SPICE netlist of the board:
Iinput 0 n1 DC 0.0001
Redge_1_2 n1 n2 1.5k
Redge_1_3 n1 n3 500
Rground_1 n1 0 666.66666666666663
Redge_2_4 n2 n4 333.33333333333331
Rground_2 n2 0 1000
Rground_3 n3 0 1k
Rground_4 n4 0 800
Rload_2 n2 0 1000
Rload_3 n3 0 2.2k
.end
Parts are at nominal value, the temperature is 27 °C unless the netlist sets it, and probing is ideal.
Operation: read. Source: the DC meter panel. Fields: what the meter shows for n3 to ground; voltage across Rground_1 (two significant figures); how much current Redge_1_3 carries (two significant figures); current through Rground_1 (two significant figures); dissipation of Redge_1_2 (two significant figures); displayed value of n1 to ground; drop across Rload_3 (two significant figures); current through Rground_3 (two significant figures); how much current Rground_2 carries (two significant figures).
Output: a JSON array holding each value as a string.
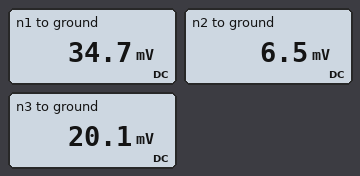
["20.1 mV", "35 mV", "29 µA", "52 µA", "530 nW", "34.7 mV", "20 mV", "20 µA", "6.5 µA"]
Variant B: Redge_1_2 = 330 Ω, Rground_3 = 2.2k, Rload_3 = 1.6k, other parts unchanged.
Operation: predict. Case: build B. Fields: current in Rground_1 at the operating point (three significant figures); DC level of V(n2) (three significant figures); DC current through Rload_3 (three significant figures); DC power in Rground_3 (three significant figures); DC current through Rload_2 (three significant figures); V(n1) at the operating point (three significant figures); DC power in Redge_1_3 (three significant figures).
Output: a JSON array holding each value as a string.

["40.8 µA", "13.9 mV", "11.0 µA", "142 nW", "13.9 µA", "27.2 mV", "182 nW"]
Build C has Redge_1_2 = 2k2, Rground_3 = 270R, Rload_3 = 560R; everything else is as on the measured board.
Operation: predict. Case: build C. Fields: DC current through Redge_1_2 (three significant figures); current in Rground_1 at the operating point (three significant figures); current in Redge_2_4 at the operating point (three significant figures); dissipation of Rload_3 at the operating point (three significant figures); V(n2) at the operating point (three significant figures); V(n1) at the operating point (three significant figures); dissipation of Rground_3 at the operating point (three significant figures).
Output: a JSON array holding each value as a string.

["11.7 µA", "44.7 µA", "3.58 µA", "113 nW", "4.06 mV", "29.8 mV", "234 nW"]
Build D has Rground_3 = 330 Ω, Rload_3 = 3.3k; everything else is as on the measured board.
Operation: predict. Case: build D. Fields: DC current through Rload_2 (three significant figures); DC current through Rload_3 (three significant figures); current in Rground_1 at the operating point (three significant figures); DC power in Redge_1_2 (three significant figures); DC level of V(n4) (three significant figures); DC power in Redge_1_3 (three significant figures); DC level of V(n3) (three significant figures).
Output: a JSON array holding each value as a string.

["5.71 µA", "3.45 µA", "45.6 µA", "406 nW", "4.03 mV", "721 nW", "11.4 mV"]
